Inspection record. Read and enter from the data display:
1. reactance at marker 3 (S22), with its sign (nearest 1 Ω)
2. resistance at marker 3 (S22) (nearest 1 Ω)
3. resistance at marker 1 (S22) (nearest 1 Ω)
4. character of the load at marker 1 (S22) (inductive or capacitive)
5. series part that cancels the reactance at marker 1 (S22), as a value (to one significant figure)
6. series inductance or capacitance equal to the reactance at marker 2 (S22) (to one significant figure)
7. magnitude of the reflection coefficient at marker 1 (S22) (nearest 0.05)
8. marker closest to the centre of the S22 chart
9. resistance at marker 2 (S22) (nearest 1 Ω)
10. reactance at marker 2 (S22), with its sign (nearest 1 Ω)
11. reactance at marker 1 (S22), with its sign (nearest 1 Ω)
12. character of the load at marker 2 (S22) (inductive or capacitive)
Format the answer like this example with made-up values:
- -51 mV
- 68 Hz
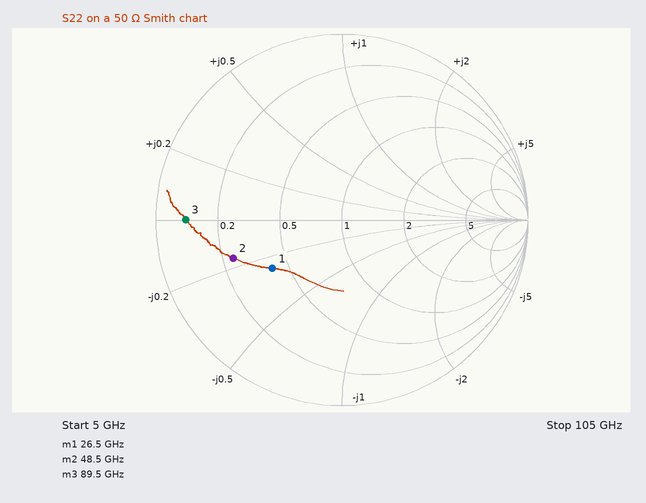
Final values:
- 0 Ω
- 4 Ω
- 20 Ω
- capacitive
- 80 pH
- 400 fF
- 0.45
- marker 1
- 12 Ω
- -8 Ω
- -13 Ω
- capacitive
